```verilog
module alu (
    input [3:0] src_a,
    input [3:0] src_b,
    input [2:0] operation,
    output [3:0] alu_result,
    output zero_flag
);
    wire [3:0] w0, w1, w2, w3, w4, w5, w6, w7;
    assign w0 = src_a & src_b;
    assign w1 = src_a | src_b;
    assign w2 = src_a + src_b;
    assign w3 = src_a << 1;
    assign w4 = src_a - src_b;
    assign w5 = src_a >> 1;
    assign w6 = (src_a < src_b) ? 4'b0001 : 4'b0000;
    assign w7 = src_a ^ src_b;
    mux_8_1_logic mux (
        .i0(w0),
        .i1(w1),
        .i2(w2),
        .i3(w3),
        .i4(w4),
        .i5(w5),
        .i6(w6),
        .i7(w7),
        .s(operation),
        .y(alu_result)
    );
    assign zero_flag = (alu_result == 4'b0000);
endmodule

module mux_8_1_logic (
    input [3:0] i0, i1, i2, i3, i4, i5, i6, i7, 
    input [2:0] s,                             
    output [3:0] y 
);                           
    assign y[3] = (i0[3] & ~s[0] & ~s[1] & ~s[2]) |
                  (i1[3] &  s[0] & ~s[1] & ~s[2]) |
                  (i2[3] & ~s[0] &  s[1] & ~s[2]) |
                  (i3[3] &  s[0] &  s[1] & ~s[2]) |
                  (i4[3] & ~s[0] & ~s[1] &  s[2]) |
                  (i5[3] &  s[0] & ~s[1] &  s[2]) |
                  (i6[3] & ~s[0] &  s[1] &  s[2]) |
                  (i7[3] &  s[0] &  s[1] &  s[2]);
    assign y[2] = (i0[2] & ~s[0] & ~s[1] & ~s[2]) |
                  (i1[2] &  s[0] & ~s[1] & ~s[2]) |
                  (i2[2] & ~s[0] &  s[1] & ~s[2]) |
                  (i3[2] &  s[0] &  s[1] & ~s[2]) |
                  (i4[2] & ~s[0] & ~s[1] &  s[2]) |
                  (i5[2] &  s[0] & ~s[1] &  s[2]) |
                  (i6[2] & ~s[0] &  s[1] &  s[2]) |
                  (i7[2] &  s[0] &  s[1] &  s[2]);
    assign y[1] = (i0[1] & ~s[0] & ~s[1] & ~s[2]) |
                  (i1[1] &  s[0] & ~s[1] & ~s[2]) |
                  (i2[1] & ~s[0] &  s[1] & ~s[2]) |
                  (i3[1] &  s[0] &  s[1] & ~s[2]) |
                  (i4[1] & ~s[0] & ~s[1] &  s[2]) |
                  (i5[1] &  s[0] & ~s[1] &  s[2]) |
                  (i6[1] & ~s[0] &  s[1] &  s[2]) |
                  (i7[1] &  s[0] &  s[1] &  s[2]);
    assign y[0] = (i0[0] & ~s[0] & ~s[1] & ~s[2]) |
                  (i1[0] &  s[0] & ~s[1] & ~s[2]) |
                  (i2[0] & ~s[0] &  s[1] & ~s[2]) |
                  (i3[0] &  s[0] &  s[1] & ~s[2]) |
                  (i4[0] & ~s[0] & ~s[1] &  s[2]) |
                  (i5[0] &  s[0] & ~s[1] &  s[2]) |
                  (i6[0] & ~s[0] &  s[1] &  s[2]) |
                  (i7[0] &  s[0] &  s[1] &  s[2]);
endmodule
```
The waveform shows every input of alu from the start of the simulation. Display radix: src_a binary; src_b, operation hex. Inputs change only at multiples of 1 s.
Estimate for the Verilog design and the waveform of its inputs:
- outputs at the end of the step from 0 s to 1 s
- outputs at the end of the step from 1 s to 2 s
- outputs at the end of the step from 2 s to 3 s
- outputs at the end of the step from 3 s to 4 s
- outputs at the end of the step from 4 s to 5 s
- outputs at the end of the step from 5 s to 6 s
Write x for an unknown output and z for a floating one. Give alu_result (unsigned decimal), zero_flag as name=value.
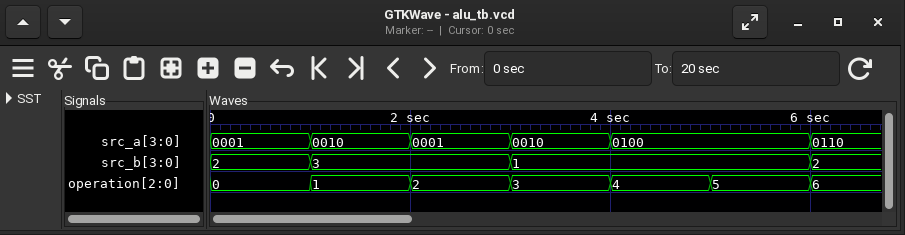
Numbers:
alu_result=0, zero_flag=1
alu_result=3, zero_flag=0
alu_result=4, zero_flag=0
alu_result=4, zero_flag=0
alu_result=3, zero_flag=0
alu_result=2, zero_flag=0
